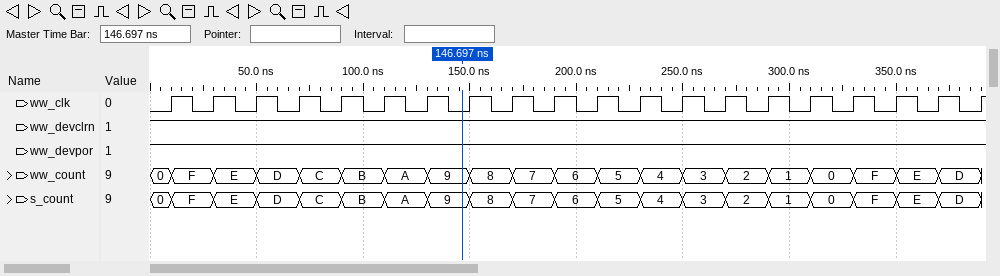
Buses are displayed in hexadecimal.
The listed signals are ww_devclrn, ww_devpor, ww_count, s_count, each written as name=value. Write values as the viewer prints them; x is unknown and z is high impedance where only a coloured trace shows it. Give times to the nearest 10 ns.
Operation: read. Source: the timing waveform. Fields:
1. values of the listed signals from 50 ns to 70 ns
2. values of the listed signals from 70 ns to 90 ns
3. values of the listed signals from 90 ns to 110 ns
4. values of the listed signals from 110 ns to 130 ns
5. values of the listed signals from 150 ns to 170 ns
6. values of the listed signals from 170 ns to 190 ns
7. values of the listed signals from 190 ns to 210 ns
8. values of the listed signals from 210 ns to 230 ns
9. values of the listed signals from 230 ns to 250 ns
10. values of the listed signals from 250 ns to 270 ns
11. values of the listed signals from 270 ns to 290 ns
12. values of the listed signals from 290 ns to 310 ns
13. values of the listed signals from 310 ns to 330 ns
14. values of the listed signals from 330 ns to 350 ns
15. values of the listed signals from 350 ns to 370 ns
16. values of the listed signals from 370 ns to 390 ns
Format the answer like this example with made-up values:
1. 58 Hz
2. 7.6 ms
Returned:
1. ww_devclrn=1, ww_devpor=1, ww_count=D, s_count=D
2. ww_devclrn=1, ww_devpor=1, ww_count=C, s_count=C
3. ww_devclrn=1, ww_devpor=1, ww_count=B, s_count=B
4. ww_devclrn=1, ww_devpor=1, ww_count=A, s_count=A
5. ww_devclrn=1, ww_devpor=1, ww_count=8, s_count=8
6. ww_devclrn=1, ww_devpor=1, ww_count=7, s_count=7
7. ww_devclrn=1, ww_devpor=1, ww_count=6, s_count=6
8. ww_devclrn=1, ww_devpor=1, ww_count=5, s_count=5
9. ww_devclrn=1, ww_devpor=1, ww_count=4, s_count=4
10. ww_devclrn=1, ww_devpor=1, ww_count=3, s_count=3
11. ww_devclrn=1, ww_devpor=1, ww_count=2, s_count=2
12. ww_devclrn=1, ww_devpor=1, ww_count=1, s_count=1
13. ww_devclrn=1, ww_devpor=1, ww_count=0, s_count=0
14. ww_devclrn=1, ww_devpor=1, ww_count=F, s_count=F
15. ww_devclrn=1, ww_devpor=1, ww_count=E, s_count=E
16. ww_devclrn=1, ww_devpor=1, ww_count=D, s_count=D
